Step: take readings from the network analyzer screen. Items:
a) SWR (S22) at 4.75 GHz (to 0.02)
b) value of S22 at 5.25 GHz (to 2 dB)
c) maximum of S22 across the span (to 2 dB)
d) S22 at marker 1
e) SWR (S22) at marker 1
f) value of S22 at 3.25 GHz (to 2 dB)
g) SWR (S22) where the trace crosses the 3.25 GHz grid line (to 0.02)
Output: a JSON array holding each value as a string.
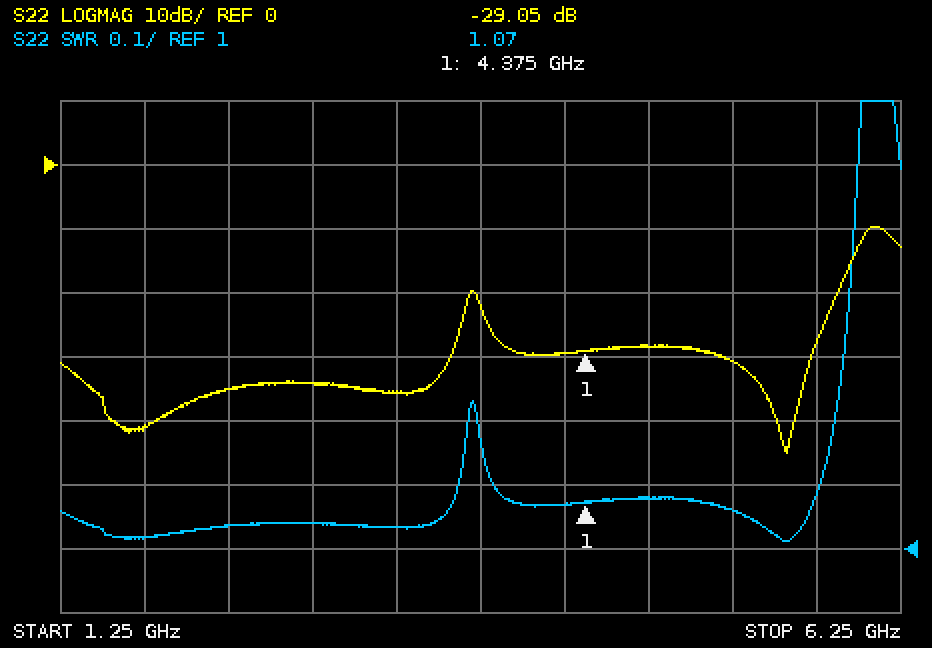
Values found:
["1.08", "-30 dB", "-10 dB", "-29.05 dB", "1.07", "-36 dB", "1.04"]
